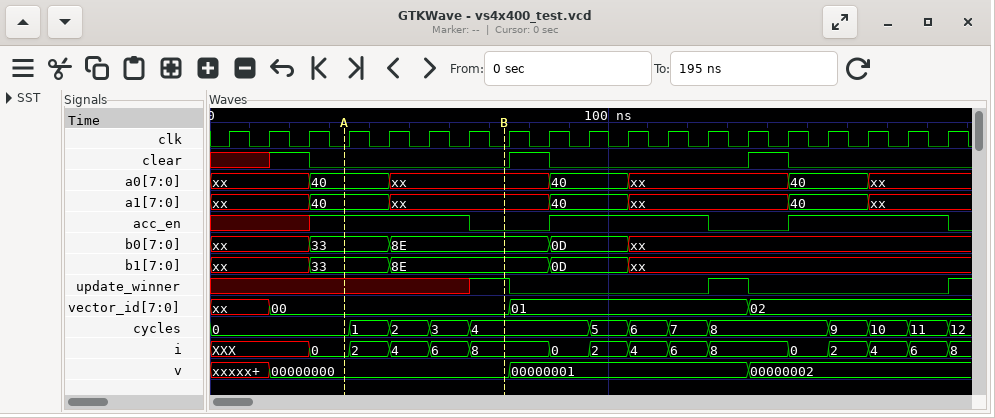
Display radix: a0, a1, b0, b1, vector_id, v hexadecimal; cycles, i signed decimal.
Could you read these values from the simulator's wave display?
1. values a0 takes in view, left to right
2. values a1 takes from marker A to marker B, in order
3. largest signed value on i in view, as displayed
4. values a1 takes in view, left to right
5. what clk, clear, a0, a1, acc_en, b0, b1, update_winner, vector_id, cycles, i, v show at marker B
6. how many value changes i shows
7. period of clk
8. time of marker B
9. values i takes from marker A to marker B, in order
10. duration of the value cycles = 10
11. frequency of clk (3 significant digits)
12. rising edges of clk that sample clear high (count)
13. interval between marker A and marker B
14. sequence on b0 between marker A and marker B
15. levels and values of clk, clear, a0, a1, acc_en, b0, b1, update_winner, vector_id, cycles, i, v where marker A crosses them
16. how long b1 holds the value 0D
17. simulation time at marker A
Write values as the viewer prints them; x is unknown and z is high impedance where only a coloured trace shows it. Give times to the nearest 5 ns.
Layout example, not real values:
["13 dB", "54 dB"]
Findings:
["xx, 40, xx, 40, xx, 40, xx", "40, xx", "8", "xx, 40, xx, 40, xx, 40, xx", "clk=0, clear=0, a0=xx, a1=xx, acc_en=0, b0=8E, b1=8E, update_winner=1, vector_id=00, cycles=4, i=8, v=00000000", "15", "10 ns", "75 ns", "0, 2, 4, 6, 8", "10 ns", "100 MHz", "3", "40 ns", "33, 8E", "clk=0, clear=0, a0=40, a1=40, acc_en=1, b0=33, b1=33, update_winner=x, vector_id=00, cycles=0, i=0, v=00000000", "20 ns", "35 ns"]
